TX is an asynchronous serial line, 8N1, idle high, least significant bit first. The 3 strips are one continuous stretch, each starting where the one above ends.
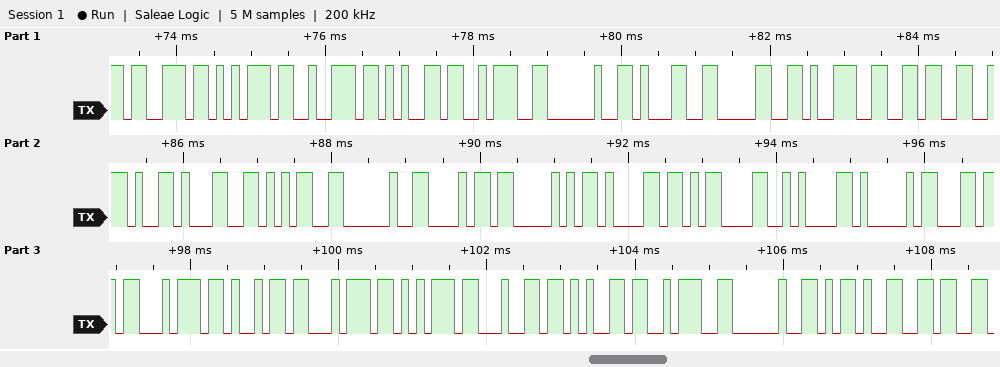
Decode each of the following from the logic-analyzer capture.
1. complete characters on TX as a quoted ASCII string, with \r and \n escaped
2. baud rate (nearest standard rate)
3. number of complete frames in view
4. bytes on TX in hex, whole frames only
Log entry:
"sure: 1096.15 hPa\r\nAltitude: -6"
9600 baud
31
73 75 72 65 3A 20 31 30 39 36 2E 31 35 20 68 50 61 0D 0A 41 6C 74 69 74 75 64 65 3A 20 2D 36
